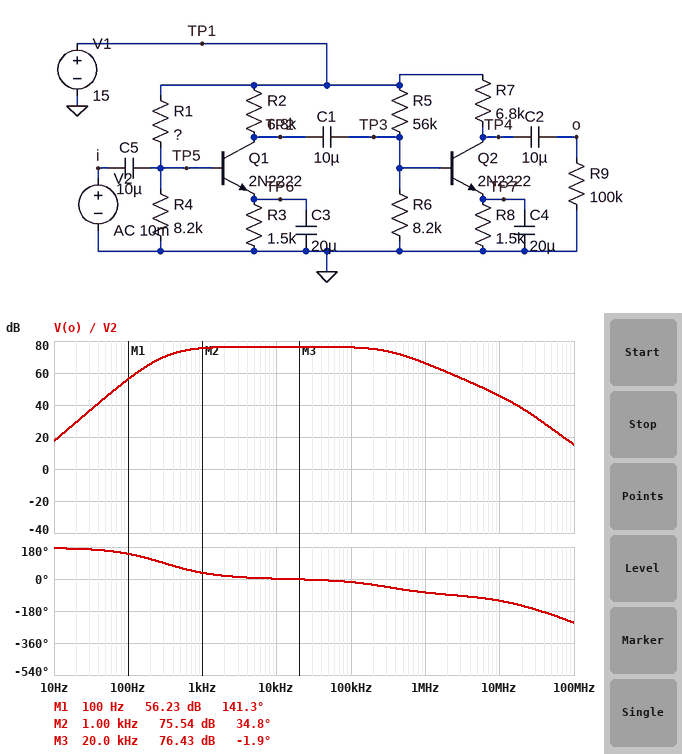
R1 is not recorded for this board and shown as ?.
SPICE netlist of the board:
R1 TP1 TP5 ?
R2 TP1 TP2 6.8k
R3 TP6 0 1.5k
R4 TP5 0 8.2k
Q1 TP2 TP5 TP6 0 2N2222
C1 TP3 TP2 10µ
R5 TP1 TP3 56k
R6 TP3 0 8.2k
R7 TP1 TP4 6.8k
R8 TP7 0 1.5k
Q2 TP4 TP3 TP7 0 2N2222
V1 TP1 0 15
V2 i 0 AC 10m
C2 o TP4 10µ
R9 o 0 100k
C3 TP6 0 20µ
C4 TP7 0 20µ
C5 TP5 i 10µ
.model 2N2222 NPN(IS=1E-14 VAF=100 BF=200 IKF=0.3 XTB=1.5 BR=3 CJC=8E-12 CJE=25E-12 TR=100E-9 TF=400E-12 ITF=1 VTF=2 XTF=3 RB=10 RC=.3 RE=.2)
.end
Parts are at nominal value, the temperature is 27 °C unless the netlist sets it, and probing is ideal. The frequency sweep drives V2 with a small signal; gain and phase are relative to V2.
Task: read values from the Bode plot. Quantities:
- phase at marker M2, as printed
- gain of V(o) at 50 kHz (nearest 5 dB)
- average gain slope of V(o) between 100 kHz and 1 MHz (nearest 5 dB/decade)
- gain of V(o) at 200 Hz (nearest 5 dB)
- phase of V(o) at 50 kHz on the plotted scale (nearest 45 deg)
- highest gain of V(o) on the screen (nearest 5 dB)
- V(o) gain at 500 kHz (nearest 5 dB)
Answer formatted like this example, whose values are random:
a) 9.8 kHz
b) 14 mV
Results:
a) 34.8 deg
b) 75 dB
c) -10 dB/decade
d) 65 dB
e) 0 deg
f) 75 dB
g) 70 dB
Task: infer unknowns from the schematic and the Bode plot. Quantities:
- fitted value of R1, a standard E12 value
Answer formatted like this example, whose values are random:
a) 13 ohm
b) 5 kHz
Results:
a) 27 kΩ
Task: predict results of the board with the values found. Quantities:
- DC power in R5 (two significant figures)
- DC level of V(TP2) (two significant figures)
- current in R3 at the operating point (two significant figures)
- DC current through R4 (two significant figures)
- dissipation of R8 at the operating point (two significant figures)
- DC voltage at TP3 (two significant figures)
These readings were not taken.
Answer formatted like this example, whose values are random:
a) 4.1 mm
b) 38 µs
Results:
a) 3.1 mW
b) 2.8 V
c) 1.8 mA
d) 410 µA
e) 1.0 mW
f) 1.9 V
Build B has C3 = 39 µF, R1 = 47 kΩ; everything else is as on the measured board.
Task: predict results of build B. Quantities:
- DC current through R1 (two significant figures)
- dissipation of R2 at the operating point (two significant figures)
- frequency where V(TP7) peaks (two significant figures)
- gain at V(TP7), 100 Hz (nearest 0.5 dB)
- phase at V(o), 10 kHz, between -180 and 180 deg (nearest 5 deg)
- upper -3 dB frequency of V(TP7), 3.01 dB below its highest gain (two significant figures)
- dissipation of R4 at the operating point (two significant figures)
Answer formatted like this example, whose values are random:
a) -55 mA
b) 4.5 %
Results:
a) 270 µA
b) 7.1 mW
c) 160 Hz
d) 35.0 dB
e) -5 deg
f) 400 Hz
g) 590 µW
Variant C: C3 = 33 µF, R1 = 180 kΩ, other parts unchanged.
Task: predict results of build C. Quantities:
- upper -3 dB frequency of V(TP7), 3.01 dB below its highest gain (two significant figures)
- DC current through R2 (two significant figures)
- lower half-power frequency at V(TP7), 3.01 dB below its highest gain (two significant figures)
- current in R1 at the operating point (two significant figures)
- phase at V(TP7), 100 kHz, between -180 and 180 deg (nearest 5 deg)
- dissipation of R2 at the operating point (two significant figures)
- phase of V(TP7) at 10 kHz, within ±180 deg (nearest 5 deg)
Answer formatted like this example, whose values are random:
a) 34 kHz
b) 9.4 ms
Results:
a) 190 Hz
b) 51 µA
c) 11 Hz
d) 80 µA
e) 45 deg
f) 18 µW
g) 85 deg
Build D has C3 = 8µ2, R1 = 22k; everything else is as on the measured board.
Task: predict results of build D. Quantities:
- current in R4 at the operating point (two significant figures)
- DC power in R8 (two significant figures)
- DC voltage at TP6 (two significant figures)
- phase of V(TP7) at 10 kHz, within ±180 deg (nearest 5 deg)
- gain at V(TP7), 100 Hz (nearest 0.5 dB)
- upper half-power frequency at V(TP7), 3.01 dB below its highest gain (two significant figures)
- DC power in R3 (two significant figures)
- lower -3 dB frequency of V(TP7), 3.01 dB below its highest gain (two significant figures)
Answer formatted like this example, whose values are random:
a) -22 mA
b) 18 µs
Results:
a) 430 µA
b) 1.0 mW
c) 2.8 V
d) 95 deg
e) -3.0 dB
f) 1.0 kHz
g) 5.3 mW
h) 130 Hz
